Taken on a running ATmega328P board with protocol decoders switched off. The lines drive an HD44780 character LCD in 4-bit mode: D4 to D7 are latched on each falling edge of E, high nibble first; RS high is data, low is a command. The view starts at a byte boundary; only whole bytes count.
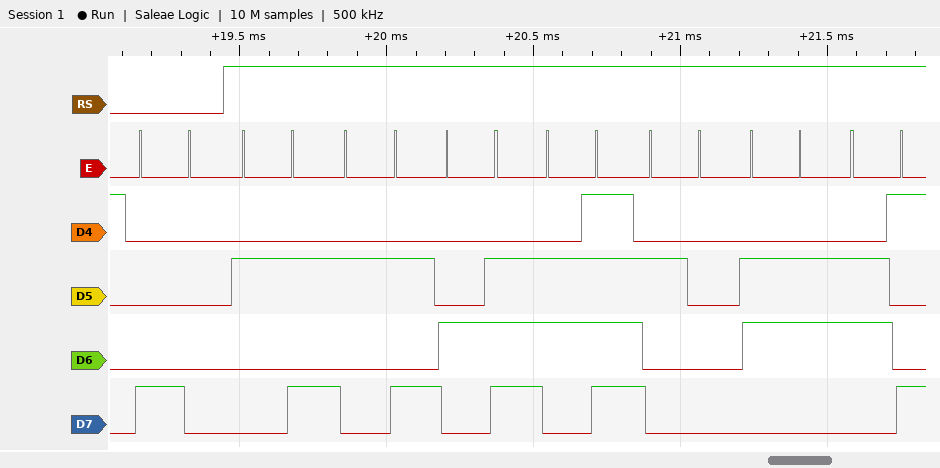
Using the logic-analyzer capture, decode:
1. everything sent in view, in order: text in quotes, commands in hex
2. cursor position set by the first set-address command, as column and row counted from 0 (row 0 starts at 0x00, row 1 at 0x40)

0x80 "**No fi"
column 0, row 0
